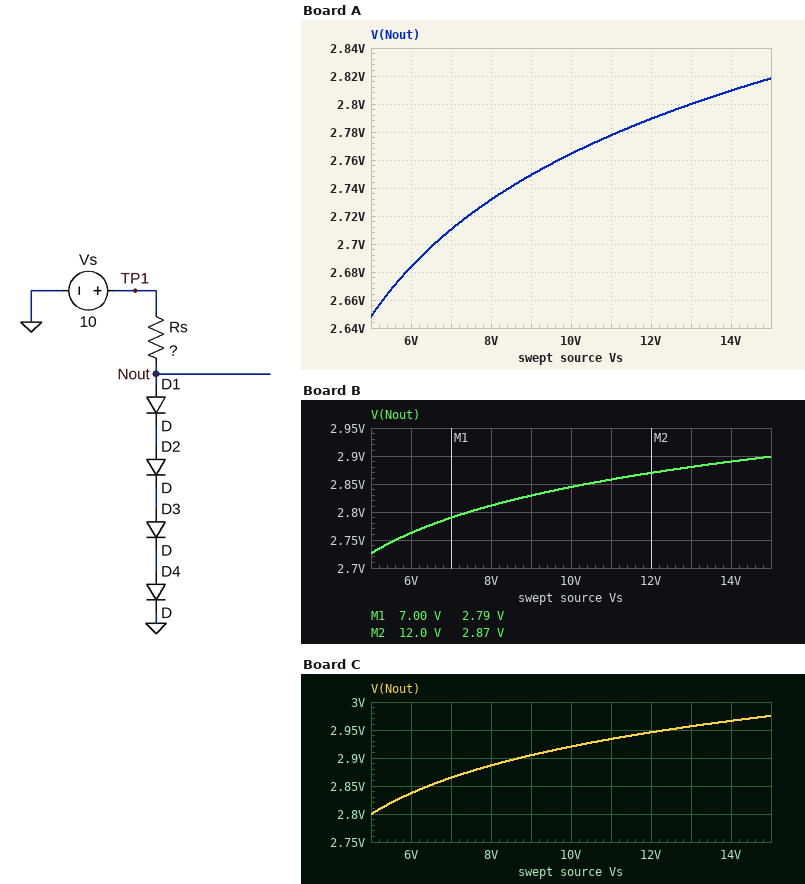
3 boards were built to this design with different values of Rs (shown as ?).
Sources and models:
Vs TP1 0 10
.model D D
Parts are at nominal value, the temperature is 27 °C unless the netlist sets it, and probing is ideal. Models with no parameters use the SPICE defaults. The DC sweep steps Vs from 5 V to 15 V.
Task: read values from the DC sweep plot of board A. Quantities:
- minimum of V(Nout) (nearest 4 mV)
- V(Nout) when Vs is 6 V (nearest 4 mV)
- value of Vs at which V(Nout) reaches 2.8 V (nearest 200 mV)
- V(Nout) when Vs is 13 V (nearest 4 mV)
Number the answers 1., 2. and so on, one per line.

1. 2.648 V
2. 2.684 V
3. 13.0 V
4. 2.800 V
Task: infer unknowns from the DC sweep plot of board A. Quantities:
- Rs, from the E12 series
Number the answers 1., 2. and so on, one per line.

1. 1.8 kΩ
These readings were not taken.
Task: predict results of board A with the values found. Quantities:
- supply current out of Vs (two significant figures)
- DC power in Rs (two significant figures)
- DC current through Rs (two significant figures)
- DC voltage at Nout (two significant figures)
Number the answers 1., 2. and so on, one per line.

1. 4.0 mA
2. 29 mW
3. 4.0 mA
4. 2.8 V
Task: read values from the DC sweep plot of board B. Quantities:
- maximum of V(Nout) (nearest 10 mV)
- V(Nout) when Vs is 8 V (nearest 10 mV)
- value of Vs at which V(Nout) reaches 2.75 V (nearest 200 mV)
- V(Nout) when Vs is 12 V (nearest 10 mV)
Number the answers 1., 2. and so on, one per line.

1. 2.90 V
2. 2.81 V
3. 5.6 V
4. 2.87 V
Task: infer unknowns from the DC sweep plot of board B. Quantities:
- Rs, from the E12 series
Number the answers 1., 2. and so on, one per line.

1. 820 Ω
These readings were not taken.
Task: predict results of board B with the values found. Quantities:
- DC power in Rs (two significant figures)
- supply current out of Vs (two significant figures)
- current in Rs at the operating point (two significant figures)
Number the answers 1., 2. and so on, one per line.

1. 62 mW
2. 8.7 mA
3. 8.7 mA
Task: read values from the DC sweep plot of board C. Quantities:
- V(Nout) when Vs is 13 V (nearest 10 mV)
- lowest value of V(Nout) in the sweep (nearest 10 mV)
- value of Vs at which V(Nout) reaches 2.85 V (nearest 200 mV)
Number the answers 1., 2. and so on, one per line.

1. 2.96 V
2. 2.80 V
3. 6.4 V
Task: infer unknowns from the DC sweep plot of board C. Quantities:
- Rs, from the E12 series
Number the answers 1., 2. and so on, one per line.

1. 390 Ω
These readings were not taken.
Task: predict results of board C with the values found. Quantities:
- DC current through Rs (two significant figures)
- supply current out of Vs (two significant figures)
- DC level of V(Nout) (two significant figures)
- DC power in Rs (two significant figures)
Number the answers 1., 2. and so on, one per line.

1. 18 mA
2. 18 mA
3. 2.9 V
4. 130 mW
